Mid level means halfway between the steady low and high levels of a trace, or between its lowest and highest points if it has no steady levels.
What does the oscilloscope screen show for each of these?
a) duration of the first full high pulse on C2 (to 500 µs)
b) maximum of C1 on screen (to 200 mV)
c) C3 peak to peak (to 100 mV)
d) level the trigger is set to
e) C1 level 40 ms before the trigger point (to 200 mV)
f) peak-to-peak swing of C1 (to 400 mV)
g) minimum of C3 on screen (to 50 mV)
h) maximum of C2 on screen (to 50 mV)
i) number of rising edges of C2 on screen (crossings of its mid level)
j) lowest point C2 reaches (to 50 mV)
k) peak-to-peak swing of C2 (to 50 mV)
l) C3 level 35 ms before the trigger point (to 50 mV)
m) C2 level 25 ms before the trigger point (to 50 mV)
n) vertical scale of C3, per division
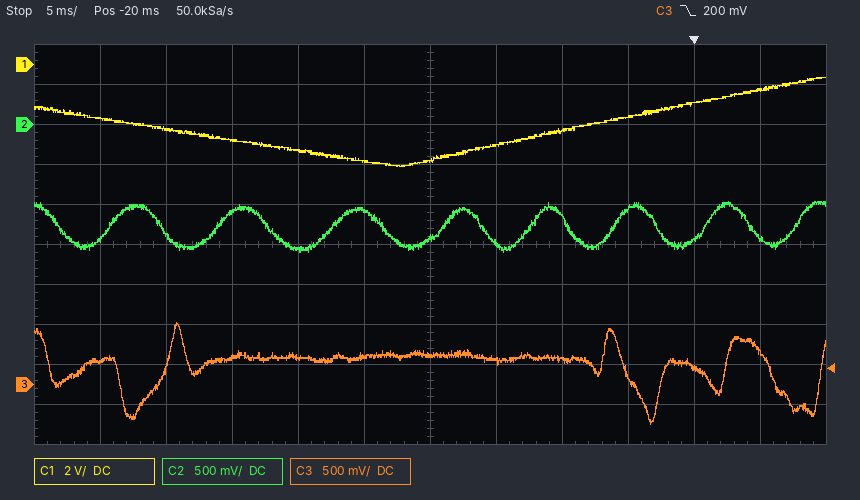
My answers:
4.0 ms
-600 mV
1.30 V
200 mV
-3.2 V
4.4 V
-500 mV
-950 mV
8
-1.60 V
650 mV
350 mV
-1.05 V
500 mV
